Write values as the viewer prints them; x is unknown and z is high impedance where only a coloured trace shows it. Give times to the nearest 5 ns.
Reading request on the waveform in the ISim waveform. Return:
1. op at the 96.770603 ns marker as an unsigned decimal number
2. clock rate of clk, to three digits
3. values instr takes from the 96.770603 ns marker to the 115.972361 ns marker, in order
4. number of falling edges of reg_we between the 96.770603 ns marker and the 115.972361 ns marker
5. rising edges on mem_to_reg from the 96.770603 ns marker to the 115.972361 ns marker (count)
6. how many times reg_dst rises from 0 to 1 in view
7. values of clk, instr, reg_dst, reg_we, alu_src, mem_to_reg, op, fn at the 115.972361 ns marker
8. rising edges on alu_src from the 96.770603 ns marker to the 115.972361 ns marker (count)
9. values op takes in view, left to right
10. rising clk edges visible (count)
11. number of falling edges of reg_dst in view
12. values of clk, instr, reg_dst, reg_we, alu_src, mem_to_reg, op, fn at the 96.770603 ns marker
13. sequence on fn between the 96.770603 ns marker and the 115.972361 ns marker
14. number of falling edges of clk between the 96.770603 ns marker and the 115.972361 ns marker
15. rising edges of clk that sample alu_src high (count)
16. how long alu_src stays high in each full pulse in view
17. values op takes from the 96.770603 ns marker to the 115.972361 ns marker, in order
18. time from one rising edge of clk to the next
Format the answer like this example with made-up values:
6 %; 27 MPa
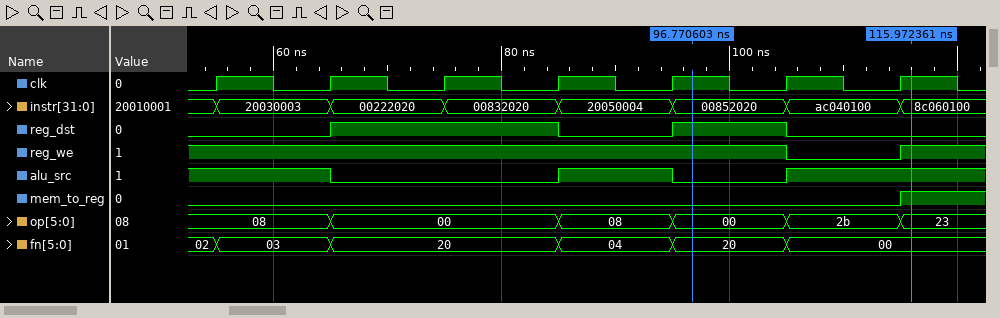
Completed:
0; 100 MHz; 00852020, ac040100, 8c060100; 1; 1; 2; clk=1, instr=8c060100, reg_dst=0, reg_we=1, alu_src=1, mem_to_reg=1, op=23, fn=00; 1; 08, 00, 08, 00, 2b, 23; 7; 2; clk=1, instr=00852020, reg_dst=1, reg_we=1, alu_src=0, mem_to_reg=0, op=00, fn=20; 20, 00; 2; 4; 10 ns; 00, 2b, 23; 10 ns
